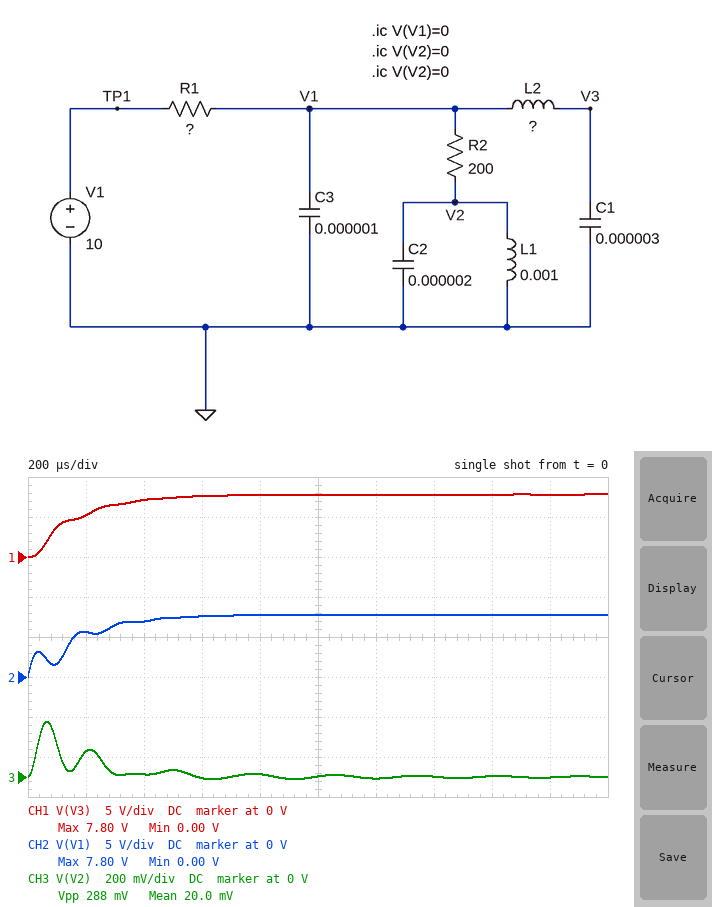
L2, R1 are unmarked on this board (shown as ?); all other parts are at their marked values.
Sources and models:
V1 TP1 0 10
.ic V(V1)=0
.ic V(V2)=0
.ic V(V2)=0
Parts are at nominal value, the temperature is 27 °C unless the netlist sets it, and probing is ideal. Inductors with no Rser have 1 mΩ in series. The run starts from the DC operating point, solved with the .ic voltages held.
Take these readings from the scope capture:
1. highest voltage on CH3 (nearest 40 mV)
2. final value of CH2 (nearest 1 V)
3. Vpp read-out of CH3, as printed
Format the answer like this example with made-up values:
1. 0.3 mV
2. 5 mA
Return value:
1. 280 mV
2. 8 V
3. 288 mV
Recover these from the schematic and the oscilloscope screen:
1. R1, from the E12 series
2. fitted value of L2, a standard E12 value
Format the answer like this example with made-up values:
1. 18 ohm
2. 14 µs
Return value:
1. 56 Ω
2. 680 µH
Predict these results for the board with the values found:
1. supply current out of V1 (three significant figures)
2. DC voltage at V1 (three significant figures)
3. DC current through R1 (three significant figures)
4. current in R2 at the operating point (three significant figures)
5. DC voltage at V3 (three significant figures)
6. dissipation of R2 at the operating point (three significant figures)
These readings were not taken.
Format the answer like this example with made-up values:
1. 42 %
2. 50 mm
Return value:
1. 39.1 mA
2. 7.81 V
3. 39.1 mA
4. 39.1 mA
5. 7.81 V
6. 305 mW
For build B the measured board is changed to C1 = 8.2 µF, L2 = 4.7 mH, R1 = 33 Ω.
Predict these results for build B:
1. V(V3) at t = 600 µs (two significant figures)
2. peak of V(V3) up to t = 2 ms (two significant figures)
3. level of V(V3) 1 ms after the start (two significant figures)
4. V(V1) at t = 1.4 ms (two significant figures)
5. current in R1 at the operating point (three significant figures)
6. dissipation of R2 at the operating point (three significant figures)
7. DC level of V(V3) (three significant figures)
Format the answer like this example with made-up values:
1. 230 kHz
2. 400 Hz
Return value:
1. 8.8 V
2. 9.2 V
3. 8.9 V
4. 8.6 V
5. 42.9 mA
6. 368 mW
7. 8.58 V
